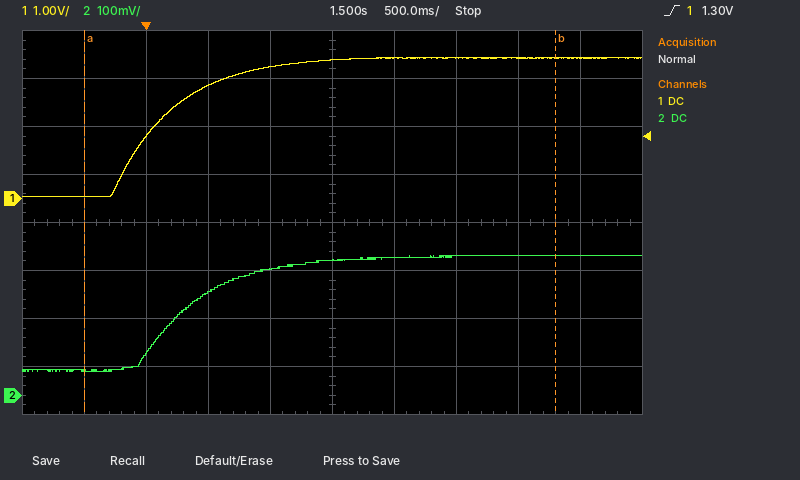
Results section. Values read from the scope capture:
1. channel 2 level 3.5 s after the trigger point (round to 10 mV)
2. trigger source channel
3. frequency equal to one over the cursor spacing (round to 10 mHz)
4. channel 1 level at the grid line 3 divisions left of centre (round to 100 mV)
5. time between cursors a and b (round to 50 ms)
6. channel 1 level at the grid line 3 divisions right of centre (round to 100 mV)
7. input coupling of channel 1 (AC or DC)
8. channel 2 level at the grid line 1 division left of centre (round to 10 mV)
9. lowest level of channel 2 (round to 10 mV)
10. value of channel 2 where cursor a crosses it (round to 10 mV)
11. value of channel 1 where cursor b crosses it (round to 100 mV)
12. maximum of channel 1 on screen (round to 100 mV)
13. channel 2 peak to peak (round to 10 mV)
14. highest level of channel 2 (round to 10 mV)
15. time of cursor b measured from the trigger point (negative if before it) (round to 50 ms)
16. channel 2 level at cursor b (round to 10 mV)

290 mV
channel 1
260 mHz
1.3 V
3.80 s
2.9 V
DC
260 mV
50 mV
50 mV
2.9 V
2.9 V
240 mV
290 mV
+3.30 s
290 mV
